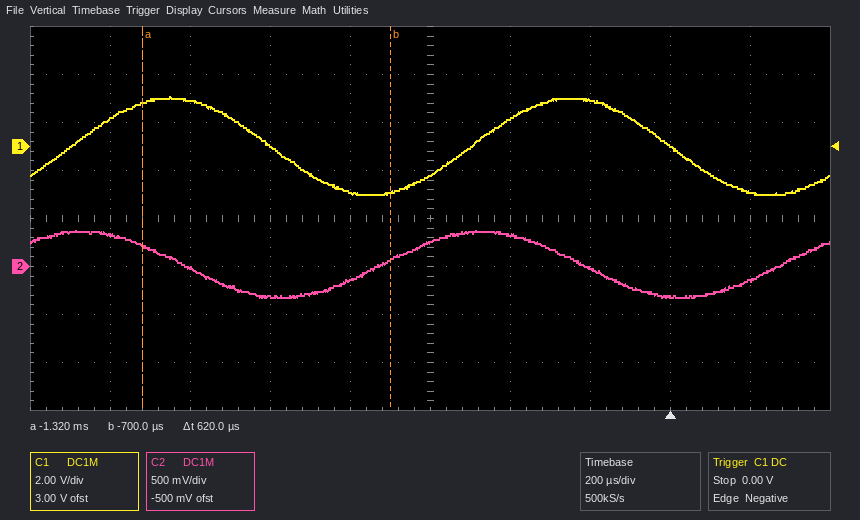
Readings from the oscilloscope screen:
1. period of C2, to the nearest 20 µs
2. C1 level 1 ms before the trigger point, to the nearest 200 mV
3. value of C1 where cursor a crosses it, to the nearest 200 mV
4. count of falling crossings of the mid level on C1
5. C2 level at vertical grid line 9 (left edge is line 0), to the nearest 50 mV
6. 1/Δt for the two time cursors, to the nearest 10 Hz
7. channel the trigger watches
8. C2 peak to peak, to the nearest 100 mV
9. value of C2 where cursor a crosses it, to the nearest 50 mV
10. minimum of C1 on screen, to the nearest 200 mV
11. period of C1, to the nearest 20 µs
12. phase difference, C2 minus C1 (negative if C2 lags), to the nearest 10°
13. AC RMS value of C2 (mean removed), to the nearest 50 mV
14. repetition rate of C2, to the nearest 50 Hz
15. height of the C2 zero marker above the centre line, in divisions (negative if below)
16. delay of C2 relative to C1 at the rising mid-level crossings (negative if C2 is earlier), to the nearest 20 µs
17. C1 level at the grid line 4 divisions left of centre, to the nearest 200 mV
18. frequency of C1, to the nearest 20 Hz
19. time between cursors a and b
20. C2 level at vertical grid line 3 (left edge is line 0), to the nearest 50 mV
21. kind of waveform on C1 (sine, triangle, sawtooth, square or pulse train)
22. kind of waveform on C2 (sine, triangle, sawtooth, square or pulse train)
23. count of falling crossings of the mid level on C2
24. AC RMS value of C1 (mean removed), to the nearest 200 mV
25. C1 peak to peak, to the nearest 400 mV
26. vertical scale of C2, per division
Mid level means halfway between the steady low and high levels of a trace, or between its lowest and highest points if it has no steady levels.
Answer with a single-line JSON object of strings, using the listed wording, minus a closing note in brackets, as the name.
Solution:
{"period of C2, to the nearest 20 µs": "1.00 ms", "C1 level 1 ms before the trigger point, to the nearest 200 mV": "0.0 V", "value of C1 where cursor a crosses it, to the nearest 200 mV": "1.8 V", "count of falling crossings of the mid level on C1": "2", "C2 level at vertical grid line 9 (left edge is line 0), to the nearest 50 mV": "-150 mV", "1/Δt for the two time cursors, to the nearest 10 Hz": "1.61 kHz", "channel the trigger watches": "C1", "C2 peak to peak, to the nearest 100 mV": "700 mV", "value of C2 where cursor a crosses it, to the nearest 50 mV": "200 mV", "minimum of C1 on screen, to the nearest 200 mV": "-2.0 V", "period of C1, to the nearest 20 µs": "1.00 ms", "phase difference, C2 minus C1 (negative if C2 lags), to the nearest 10°": "+80°", "AC RMS value of C2 (mean removed), to the nearest 50 mV": "250 mV", "repetition rate of C2, to the nearest 50 Hz": "1.00 kHz", "height of the C2 zero marker above the centre line, in divisions": "-1.0 div", "delay of C2 relative to C1 at the rising mid-level crossings (negative if C2 is earlier), to the nearest 20 µs": "-220 µs", "C1 level at the grid line 4 divisions left of centre, to the nearest 200 mV": "1.2 V", "frequency of C1, to the nearest 20 Hz": "1.00 kHz", "time between cursors a and b": "620 µs", "C2 level at vertical grid line 3 (left edge is line 0), to the nearest 50 mV": "-300 mV", "kind of waveform on C1": "sine", "kind of waveform on C2": "sine", "count of falling crossings of the mid level on C2": "2", "AC RMS value of C1 (mean removed), to the nearest 200 mV": "1.4 V", "C1 peak to peak, to the nearest 400 mV": "4.0 V", "vertical scale of C2, per division": "500 mV"}
